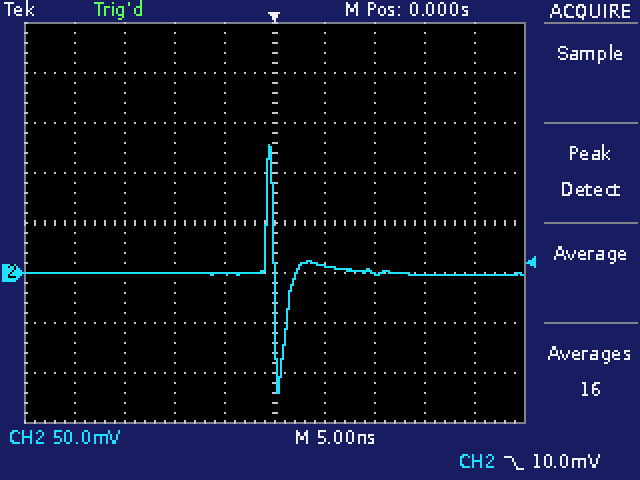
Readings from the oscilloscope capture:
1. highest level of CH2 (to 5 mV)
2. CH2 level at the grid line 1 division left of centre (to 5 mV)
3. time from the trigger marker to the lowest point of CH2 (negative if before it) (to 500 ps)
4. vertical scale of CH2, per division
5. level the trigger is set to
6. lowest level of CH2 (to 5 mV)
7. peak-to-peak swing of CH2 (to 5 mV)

130 mV
0 mV
+500 ps
50 mV
10.0 mV
-120 mV
250 mV
